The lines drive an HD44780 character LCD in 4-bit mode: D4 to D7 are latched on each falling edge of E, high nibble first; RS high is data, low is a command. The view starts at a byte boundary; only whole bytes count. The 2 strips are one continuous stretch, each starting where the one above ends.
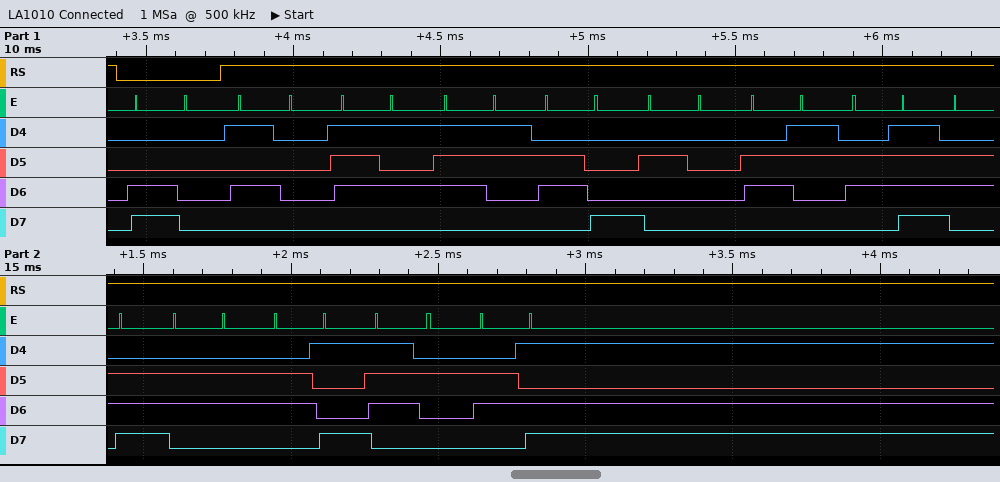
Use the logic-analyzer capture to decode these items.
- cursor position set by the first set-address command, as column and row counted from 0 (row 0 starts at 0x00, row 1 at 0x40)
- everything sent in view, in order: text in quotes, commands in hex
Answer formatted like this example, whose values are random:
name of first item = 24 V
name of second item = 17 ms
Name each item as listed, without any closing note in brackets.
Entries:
cursor position set by the first set-address command, as column and row counted from 0 = column 0, row 1
everything sent in view, in order: text in quotes, commands in hex = 0xC0 "Push confirm"
